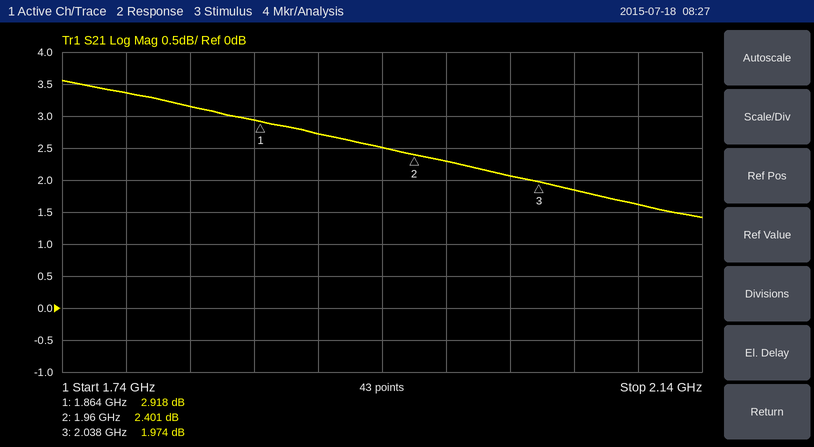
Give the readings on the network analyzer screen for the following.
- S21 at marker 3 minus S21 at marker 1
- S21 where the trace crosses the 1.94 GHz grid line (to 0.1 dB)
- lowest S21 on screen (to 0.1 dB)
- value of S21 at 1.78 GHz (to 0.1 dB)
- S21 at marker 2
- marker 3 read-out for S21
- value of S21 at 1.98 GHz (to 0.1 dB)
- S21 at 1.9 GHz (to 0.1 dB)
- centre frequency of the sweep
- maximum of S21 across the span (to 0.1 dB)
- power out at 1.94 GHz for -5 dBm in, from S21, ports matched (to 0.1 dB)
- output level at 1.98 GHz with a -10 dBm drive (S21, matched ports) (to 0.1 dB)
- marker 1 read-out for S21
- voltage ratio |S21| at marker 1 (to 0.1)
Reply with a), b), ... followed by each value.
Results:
a) -0.944 dB
b) 2.5 dB
c) 1.4 dB
d) 3.4 dB
e) 2.401 dB
f) 1.974 dB
g) 2.3 dB
h) 2.7 dB
i) 1.94 GHz
j) 3.6 dB
k) -2.5 dBm
l) -7.7 dBm
m) 2.918 dB
n) 1.4
